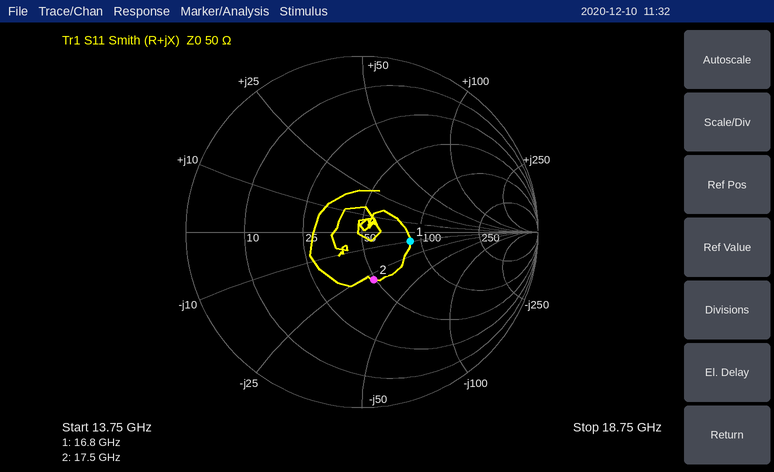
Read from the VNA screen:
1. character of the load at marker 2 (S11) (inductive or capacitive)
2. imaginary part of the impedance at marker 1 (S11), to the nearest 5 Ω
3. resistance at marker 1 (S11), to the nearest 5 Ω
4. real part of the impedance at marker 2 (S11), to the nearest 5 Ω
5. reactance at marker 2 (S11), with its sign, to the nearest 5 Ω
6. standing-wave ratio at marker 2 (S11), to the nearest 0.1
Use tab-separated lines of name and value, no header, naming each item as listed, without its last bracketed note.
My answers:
character of the load at marker 2 (S11)	capacitive
imaginary part of the impedance at marker 1 (S11), to the nearest 5 Ω	-10 Ω
resistance at marker 1 (S11), to the nearest 5 Ω	85 Ω
real part of the impedance at marker 2 (S11), to the nearest 5 Ω	50 Ω
reactance at marker 2 (S11), with its sign, to the nearest 5 Ω	-30 Ω
standing-wave ratio at marker 2 (S11), to the nearest 0.1	1.8
